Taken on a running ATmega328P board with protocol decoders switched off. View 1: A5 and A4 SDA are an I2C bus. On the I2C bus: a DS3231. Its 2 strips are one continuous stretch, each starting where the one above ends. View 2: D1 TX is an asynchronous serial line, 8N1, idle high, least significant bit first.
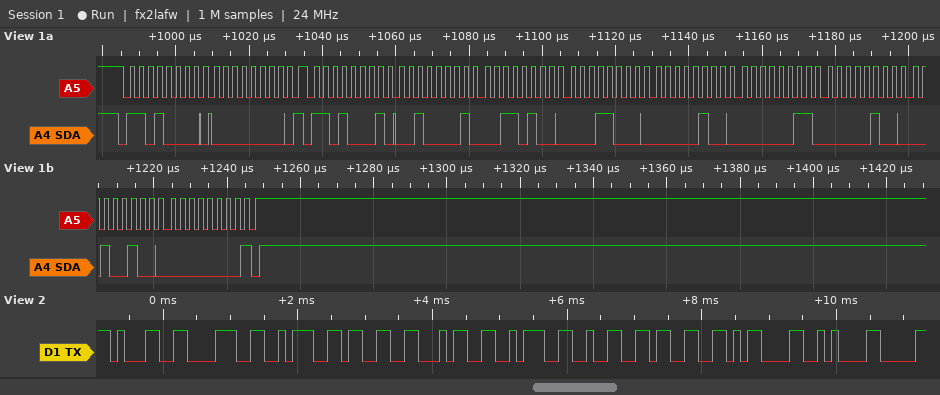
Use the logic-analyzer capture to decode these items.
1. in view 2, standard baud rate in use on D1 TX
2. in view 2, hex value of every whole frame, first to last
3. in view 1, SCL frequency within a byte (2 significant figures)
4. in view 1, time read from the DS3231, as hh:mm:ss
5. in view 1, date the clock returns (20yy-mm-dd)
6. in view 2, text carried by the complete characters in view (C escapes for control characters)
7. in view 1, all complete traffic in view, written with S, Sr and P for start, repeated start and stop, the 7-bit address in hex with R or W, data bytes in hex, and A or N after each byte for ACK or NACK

9600 baud
0x31 0x38 0x3A 0x33 0x34 0x3A 0x32 0x33 0x0D 0x0A
400 kHz
18:34:21
2024-04-03
"18:34:23\r\n"
S 68W A 00 A Sr 68R A 21 A 34 A 18 A 04 A 03 A 04 A 24 A 00 N P
